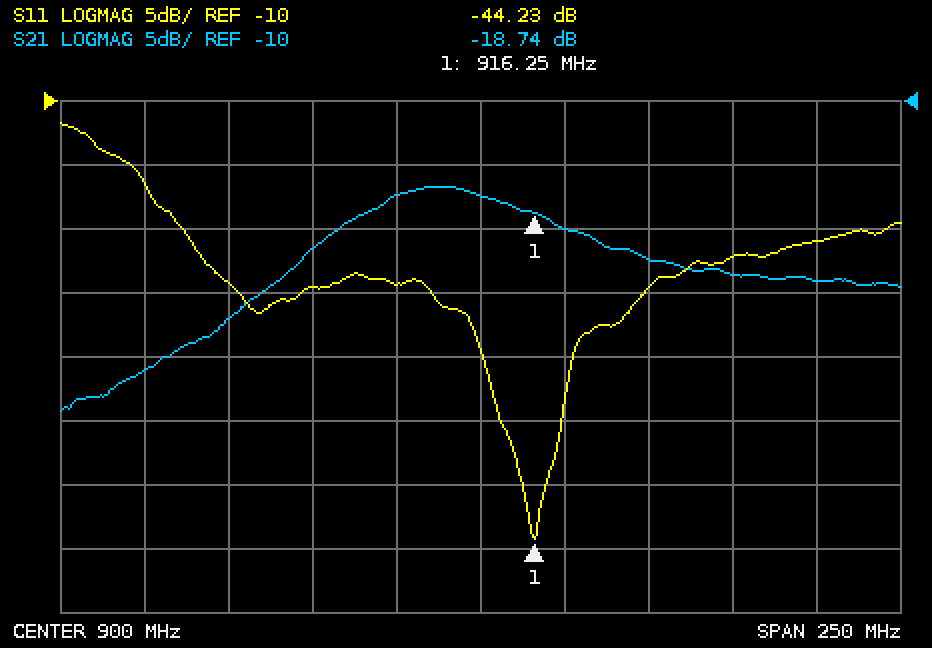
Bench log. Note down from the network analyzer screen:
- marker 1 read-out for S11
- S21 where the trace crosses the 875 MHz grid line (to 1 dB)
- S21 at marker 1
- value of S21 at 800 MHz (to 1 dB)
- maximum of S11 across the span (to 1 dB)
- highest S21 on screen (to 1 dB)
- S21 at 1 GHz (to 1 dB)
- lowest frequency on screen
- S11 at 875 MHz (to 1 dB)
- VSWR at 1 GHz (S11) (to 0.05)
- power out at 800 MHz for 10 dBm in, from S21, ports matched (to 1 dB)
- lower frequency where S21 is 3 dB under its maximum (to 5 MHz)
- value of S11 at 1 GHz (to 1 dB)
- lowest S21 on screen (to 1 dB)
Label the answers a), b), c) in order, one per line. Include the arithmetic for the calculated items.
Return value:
a) -44.23 dB
b) -17 dB
c) -18.74 dB
d) -31 dB
e) -12 dB
f) -17 dB
g) -24 dB
h) 775 MHz
i) -24 dB
j) |Γ| = 10^(-21/20) = 0.0891; VSWR = (1 + 0.0891)/(1 − 0.0891) ≈ 1.20
k) 10 dBm + (-31 dB) = -21 dBm
l) 860 MHz
m) -21 dB
n) -34 dB
